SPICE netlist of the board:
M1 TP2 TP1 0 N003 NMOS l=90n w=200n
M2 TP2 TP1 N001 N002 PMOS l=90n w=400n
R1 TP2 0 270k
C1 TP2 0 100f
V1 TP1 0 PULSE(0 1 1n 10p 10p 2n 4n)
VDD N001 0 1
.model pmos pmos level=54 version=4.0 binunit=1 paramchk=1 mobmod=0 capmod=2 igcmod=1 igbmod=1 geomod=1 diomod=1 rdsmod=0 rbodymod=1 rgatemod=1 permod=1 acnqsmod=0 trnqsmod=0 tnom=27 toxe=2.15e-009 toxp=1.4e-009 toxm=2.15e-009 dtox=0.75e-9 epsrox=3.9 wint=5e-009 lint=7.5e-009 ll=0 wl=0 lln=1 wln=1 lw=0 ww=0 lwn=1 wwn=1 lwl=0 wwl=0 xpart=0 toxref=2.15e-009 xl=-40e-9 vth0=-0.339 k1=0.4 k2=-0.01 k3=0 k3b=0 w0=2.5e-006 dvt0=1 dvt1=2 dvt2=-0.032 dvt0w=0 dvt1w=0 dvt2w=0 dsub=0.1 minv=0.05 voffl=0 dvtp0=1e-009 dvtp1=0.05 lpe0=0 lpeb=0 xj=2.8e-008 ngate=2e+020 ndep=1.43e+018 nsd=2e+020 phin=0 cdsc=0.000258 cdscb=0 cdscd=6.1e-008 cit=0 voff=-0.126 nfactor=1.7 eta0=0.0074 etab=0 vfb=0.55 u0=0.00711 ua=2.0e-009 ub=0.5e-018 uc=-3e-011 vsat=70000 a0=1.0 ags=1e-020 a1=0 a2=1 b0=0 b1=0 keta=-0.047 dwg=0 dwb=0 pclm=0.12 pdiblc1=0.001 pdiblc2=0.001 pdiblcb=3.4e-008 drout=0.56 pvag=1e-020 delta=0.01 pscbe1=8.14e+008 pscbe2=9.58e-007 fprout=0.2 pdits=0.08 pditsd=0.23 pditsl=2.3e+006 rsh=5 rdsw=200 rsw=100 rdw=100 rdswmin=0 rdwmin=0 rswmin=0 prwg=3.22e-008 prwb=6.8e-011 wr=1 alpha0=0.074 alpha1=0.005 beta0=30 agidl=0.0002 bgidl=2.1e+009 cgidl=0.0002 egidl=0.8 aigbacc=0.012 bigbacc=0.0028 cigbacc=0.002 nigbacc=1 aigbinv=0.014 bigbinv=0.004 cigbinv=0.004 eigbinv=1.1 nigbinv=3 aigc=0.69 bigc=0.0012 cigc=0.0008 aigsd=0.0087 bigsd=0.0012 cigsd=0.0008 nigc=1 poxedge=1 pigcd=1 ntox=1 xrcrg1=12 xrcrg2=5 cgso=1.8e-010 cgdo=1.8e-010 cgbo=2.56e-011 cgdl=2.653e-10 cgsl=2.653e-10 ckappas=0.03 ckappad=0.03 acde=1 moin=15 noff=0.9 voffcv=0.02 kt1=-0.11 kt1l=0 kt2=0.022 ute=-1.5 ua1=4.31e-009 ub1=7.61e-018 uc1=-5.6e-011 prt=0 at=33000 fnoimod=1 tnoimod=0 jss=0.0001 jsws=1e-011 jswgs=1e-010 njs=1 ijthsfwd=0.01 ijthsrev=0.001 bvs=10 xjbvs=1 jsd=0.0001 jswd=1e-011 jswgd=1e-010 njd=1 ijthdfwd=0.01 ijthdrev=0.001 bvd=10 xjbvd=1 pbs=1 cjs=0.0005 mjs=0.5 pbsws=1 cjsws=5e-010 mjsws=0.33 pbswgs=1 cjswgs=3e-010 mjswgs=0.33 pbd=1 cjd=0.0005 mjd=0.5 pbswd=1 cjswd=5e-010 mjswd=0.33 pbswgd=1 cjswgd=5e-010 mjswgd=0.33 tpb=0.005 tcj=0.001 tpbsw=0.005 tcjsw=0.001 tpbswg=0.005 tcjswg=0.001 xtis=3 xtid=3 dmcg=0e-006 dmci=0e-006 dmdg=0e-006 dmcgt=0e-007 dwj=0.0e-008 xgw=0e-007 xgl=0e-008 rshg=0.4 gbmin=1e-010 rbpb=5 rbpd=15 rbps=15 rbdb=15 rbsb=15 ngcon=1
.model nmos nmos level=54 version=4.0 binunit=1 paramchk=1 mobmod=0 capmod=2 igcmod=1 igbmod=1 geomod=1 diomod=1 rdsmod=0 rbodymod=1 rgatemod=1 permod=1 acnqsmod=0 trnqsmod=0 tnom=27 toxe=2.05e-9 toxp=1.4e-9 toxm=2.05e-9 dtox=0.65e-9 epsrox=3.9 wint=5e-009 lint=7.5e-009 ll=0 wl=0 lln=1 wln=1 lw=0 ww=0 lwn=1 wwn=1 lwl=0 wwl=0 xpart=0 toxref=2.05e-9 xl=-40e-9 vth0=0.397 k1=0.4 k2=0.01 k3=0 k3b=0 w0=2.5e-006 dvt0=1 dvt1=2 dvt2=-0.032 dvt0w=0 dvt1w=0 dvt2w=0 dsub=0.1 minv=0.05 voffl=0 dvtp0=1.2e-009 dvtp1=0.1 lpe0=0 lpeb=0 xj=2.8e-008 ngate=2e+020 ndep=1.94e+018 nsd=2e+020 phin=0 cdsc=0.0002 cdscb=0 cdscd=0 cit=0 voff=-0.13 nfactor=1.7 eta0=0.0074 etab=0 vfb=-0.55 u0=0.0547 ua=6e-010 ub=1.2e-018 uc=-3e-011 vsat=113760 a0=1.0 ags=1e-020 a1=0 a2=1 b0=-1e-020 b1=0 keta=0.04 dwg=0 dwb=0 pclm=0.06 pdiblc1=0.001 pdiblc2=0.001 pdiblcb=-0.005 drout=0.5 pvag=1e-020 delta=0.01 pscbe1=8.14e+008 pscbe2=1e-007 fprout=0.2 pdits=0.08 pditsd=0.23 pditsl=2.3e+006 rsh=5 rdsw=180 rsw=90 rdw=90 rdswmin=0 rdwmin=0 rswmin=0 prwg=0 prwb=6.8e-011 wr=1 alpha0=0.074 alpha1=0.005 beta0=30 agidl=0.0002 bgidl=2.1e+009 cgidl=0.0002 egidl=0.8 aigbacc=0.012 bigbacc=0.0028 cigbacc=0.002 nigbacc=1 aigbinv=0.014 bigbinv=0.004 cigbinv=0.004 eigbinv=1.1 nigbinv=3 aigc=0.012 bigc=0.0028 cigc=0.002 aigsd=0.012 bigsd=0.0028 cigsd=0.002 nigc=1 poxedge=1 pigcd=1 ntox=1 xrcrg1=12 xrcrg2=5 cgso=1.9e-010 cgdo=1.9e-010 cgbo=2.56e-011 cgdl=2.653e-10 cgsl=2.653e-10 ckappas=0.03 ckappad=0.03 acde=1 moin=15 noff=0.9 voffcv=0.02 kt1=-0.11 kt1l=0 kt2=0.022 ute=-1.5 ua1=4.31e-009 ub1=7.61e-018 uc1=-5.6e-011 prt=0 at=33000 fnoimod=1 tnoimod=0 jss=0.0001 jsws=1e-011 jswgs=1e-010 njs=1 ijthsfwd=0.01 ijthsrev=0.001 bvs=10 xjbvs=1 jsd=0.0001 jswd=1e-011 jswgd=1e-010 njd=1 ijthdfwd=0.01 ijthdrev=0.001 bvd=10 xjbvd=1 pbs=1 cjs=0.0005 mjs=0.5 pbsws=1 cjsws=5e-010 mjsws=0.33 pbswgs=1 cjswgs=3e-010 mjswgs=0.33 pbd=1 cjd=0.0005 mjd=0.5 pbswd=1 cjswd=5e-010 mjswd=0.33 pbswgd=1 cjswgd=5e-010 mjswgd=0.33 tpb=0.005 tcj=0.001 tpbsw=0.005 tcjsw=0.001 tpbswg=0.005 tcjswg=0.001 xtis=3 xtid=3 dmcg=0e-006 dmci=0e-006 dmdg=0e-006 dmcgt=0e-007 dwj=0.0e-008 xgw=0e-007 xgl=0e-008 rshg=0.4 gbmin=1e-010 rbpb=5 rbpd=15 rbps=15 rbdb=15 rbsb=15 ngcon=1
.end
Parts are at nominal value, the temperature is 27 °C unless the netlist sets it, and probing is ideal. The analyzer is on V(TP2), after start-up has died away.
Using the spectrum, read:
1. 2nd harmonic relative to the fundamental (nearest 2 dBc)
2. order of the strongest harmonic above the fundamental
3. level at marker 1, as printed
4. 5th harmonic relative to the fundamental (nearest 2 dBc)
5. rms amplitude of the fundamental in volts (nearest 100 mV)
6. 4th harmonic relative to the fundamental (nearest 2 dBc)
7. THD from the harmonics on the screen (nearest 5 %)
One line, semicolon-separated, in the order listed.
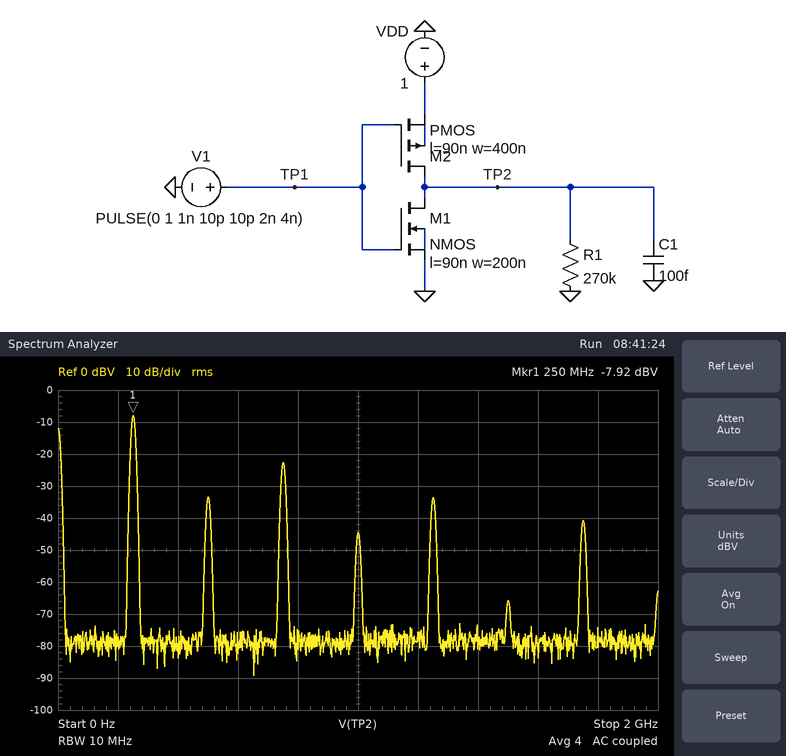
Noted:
-26 dBc; 3; -7.92 dBV; -26 dBc; 400 mV; -36 dBc; 20 %
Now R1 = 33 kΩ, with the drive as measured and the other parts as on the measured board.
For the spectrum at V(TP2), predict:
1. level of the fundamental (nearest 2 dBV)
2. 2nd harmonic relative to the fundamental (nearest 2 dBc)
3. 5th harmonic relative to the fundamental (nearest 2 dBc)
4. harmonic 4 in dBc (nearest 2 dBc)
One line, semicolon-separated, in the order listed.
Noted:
-8 dBV; -22 dBc; -24 dBc; -32 dBc
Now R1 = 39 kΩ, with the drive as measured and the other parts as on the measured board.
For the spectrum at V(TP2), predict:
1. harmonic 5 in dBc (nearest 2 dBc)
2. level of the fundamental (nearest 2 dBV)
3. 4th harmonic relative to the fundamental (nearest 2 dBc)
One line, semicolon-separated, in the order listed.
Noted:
-24 dBc; -8 dBV; -32 dBc
